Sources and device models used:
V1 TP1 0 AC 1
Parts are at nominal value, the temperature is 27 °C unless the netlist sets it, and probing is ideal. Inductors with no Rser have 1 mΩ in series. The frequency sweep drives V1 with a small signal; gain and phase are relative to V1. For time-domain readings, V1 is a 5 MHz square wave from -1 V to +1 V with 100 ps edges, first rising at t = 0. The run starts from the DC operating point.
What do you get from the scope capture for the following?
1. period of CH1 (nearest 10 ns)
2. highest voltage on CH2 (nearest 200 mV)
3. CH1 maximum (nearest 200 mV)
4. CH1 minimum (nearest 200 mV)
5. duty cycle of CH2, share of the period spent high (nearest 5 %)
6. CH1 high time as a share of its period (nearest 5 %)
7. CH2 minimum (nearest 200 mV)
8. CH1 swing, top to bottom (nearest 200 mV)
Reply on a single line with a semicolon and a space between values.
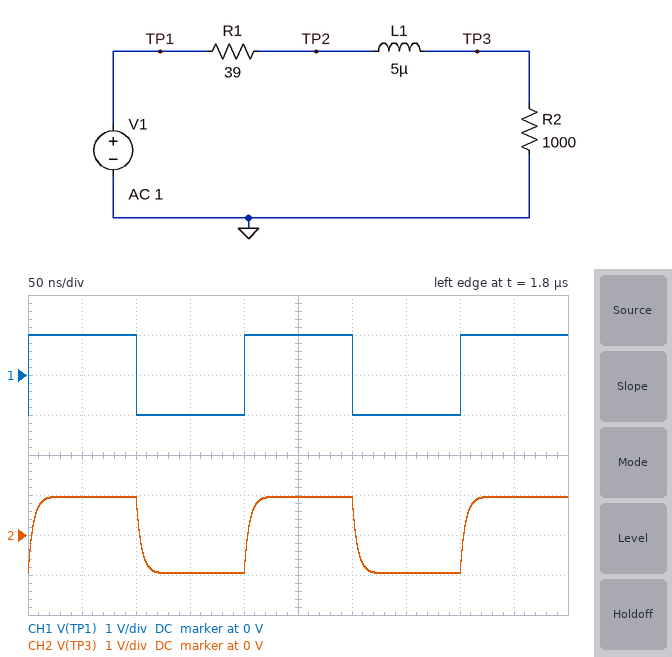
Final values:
200 ns; 1.0 V; 1.0 V; -1.0 V; 50 %; 50 %; -1.0 V; 2.0 V
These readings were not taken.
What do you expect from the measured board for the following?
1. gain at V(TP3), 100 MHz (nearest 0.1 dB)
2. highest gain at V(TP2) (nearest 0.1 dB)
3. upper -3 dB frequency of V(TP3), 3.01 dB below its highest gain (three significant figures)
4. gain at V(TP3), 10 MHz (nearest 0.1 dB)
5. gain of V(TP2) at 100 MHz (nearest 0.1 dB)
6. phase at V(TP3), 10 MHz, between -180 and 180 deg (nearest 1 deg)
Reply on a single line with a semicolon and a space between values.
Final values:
-10.4 dB; 0 dB; 33.1 MHz; -0.7 dB; 0 dB; -17 deg
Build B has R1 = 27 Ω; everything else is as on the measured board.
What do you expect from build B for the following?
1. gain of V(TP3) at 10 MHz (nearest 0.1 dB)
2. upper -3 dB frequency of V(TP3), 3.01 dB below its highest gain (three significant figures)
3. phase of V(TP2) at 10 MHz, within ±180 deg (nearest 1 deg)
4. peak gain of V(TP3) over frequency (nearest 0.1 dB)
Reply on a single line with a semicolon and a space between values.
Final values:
-0.6 dB; 32.7 MHz; 0 deg; -0.2 dB
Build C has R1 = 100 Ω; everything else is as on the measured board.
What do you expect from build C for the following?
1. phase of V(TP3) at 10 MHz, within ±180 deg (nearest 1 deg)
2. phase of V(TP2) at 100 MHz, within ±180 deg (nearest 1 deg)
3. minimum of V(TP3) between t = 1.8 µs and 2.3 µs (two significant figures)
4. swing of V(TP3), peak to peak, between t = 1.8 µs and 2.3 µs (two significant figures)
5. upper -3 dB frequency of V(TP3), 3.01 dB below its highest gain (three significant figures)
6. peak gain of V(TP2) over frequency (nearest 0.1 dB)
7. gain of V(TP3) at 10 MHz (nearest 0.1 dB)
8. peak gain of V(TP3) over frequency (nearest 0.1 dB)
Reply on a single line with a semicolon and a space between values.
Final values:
-16 deg; 2 deg; -910 mV; 1.8 V; 35.0 MHz; 0 dB; -1.2 dB; -0.8 dB
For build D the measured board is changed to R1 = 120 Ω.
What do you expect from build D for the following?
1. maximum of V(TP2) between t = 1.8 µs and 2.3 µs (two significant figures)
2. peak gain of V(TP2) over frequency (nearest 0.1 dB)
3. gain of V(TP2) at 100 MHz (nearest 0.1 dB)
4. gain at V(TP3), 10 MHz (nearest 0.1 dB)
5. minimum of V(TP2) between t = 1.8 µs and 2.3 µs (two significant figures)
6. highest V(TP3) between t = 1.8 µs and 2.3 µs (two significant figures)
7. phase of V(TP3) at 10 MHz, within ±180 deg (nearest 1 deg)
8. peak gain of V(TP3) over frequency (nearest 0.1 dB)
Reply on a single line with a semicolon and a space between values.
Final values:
1.1 V; 0 dB; -0.1 dB; -1.3 dB; -1.1 V; 890 mV; -16 deg; -1.0 dB
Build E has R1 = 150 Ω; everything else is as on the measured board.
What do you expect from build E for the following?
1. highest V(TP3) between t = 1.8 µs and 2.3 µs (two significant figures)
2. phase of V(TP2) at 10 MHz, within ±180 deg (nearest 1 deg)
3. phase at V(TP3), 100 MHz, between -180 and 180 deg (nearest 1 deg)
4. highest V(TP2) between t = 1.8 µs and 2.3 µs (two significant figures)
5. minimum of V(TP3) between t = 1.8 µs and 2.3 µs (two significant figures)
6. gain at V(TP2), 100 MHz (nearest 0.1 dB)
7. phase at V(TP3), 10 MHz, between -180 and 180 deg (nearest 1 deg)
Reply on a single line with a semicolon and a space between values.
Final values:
870 mV; 2 deg; -70 deg; 1.1 V; -870 mV; -0.1 dB; -15 deg
